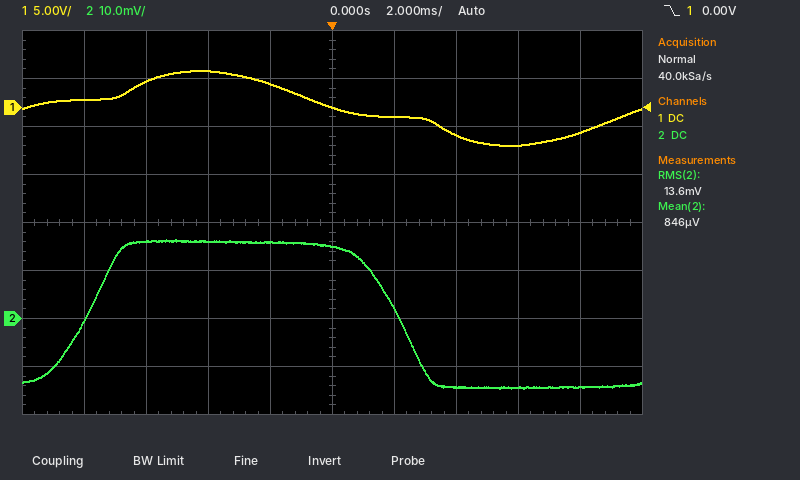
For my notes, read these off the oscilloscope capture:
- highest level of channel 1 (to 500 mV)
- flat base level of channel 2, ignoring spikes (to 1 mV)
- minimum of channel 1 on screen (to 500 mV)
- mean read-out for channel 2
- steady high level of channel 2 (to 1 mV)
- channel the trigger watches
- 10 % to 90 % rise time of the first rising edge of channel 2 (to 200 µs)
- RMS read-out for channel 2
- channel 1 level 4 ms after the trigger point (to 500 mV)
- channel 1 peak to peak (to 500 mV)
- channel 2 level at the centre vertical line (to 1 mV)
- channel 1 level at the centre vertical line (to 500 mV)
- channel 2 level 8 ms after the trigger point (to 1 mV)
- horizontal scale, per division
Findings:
4.0 V
-14 mV
-4.0 V
846 µV
16 mV
channel 1
2.2 ms
13.6 mV
-3.0 V
8.0 V
15 mV
0.0 V
-14 mV
2 ms
